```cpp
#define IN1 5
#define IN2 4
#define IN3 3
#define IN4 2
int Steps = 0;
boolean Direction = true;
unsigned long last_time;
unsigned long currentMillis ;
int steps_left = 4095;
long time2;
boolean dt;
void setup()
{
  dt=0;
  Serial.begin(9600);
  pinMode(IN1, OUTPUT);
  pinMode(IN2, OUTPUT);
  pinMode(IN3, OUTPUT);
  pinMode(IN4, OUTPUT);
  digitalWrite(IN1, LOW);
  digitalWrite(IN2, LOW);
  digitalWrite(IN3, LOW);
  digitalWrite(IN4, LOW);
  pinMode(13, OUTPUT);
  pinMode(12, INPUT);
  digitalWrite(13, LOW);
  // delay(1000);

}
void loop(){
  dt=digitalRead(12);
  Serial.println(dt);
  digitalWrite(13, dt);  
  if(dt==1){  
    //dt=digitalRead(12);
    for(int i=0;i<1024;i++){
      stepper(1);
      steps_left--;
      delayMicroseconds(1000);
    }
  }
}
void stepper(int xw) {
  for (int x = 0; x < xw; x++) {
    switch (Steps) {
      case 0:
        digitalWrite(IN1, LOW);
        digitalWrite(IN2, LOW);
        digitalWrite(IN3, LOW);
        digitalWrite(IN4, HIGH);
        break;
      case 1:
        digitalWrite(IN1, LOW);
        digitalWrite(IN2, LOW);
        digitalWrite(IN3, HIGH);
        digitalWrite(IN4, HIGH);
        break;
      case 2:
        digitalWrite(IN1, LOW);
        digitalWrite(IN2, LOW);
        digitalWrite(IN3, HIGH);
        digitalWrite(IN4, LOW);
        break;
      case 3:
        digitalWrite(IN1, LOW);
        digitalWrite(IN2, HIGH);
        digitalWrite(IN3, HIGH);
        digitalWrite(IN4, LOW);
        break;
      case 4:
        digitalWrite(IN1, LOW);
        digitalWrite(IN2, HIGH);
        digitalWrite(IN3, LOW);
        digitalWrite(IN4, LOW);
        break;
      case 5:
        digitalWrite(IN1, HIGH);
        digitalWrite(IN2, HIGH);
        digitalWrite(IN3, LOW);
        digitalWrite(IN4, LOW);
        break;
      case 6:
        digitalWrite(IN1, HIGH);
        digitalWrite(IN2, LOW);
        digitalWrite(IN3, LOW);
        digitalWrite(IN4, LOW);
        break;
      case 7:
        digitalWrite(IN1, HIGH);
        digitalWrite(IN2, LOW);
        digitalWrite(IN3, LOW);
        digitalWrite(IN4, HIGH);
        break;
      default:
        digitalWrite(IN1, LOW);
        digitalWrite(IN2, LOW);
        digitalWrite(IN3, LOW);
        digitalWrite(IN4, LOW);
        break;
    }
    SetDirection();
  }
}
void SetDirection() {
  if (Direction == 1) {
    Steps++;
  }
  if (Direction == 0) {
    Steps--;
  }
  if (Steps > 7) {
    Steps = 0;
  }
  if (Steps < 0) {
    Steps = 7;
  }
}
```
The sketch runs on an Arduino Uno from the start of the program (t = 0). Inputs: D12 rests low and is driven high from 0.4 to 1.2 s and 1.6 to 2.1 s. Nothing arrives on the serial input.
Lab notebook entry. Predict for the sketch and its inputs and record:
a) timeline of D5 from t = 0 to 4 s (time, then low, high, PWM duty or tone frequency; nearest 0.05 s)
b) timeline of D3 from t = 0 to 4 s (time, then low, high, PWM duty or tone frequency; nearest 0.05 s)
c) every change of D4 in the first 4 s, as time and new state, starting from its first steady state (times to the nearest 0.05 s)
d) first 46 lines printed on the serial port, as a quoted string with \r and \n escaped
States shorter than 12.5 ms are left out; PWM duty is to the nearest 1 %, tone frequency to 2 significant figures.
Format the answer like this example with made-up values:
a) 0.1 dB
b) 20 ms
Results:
a) 0 s low; 0.4 s tone 120 Hz; 1.45 s high; 1.6 s tone 120 Hz; 2.65 s high
b) 0 s low; 0.4 s tone 120 Hz; 1.45 s low; 1.6 s tone 120 Hz; 2.65 s low
c) 0 s low; 0.4 s tone 120 Hz; 1.45 s low; 1.6 s tone 120 Hz; 2.65 s low
d) "0\r\n0\r\n0\r\n0\r\n0\r\n0\r\n0\r\n0\r\n0\r\n0\r\n0\r\n0\r\n0\r\n0\r\n0\r\n0\r\n0\r\n0\r\n0\r\n0\r\n0\r\n0\r\n0\r\n0\r\n0\r\n0\r\n0\r\n0\r\n0\r\n0\r\n0\r\n0\r\n0\r\n0\r\n0\r\n0\r\n0\r\n0\r\n0\r\n0\r\n0\r\n0\r\n0\r\n0\r\n0\r\n0\r\n"
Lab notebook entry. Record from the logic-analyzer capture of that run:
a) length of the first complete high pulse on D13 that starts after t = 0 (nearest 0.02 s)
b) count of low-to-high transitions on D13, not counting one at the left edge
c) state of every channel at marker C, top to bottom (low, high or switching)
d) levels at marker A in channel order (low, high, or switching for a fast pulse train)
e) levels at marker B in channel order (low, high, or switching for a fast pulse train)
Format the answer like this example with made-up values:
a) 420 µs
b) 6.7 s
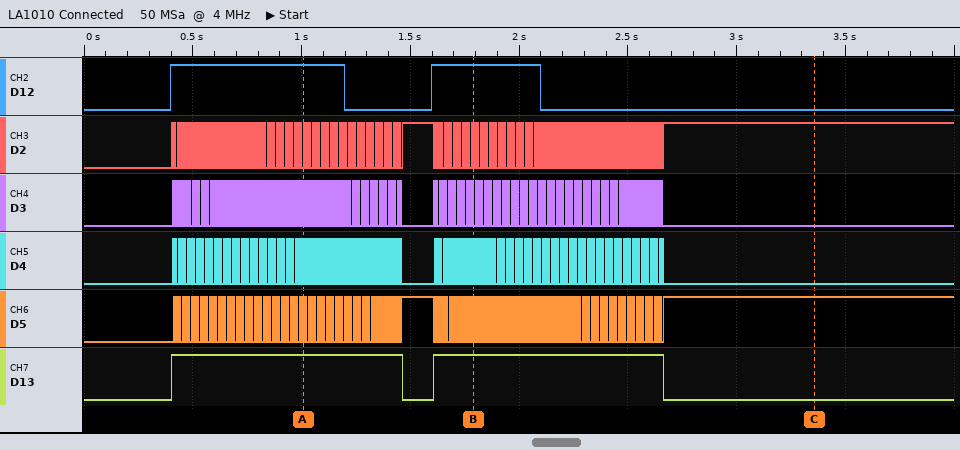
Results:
a) 1.06 s
b) 2
c) D12 low, D2 high, D3 low, D4 low, D5 high, D13 low
d) D12 high, D2 switching, D3 switching, D4 switching, D5 switching, D13 high
e) D12 high, D2 switching, D3 switching, D4 switching, D5 switching, D13 high
